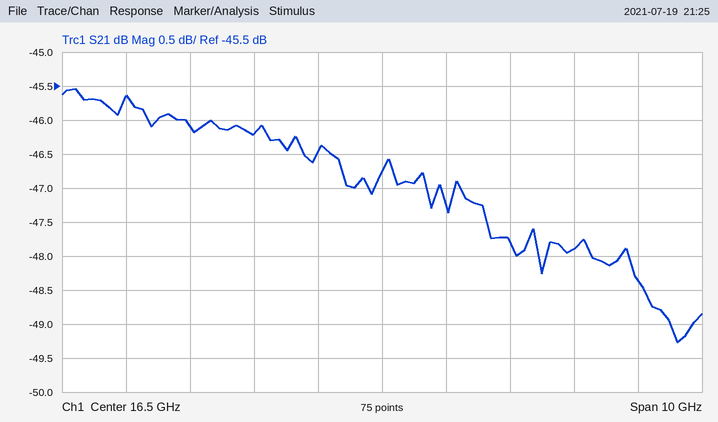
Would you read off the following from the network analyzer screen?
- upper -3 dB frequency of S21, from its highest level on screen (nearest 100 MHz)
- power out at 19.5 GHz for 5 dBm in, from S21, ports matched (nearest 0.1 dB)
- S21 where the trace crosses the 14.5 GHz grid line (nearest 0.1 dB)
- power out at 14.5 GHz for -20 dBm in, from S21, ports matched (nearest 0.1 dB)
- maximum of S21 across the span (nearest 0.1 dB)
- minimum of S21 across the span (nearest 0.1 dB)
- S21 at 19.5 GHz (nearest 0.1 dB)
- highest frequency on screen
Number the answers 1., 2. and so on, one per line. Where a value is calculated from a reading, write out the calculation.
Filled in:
1. 20.6 GHz
2. 5 dBm + (-47.9 dB) = -42.9 dBm
3. -46.2 dB
4. -20 dBm + (-46.2 dB) = -66.2 dBm
5. -45.5 dB
6. -49.3 dB
7. -47.9 dB
8. 21.5 GHz
